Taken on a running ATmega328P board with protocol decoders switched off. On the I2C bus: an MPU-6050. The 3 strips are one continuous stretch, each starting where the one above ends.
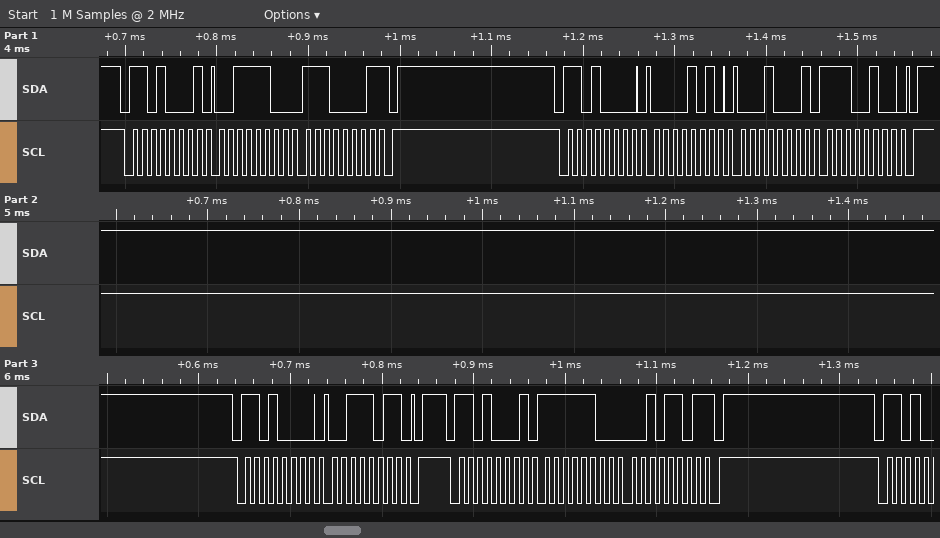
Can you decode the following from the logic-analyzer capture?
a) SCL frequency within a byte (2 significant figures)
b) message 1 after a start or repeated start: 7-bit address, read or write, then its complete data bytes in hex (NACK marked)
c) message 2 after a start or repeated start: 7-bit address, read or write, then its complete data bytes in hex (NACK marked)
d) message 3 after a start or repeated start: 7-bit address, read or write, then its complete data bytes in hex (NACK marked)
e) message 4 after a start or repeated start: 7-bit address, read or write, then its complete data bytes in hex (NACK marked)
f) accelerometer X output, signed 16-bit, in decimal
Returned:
100 kHz
0x68 read: 3C E1 NACK
0x68 write: 0A 11 E4
0x68 write: 3B
0x68 read: FC 2D NACK
-979
